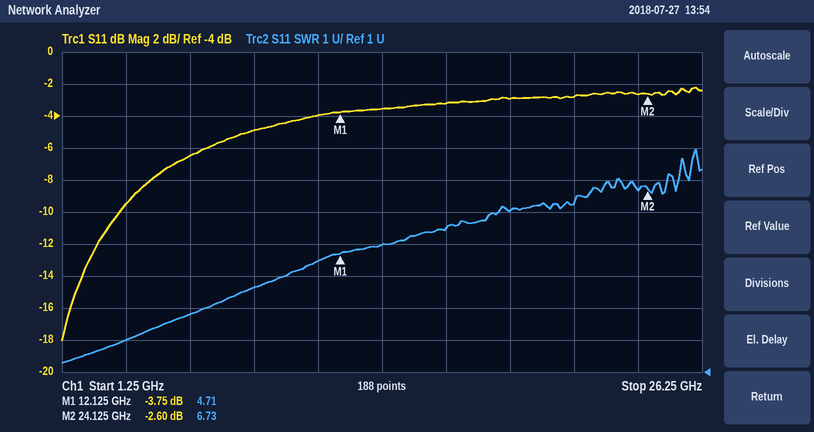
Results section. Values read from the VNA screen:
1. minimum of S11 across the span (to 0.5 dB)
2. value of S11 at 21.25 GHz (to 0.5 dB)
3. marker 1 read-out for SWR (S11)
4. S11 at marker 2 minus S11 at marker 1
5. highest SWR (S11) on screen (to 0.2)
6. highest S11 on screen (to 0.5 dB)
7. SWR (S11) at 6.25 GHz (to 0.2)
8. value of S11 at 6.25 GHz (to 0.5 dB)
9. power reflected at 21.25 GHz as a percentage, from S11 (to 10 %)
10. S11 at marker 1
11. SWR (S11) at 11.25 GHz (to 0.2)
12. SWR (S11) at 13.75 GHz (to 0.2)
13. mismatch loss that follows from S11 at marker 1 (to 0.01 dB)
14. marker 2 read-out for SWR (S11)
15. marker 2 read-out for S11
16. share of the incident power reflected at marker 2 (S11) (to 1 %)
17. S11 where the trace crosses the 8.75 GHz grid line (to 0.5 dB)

-18.0 dB
-3.0 dB
4.71
1.15 dB
8.0
-2.0 dB
2.8
-6.5 dB
50 %
-3.75 dB
4.4
5.0
2.38 dB
6.73
-2.60 dB
55 %
-5.0 dB
